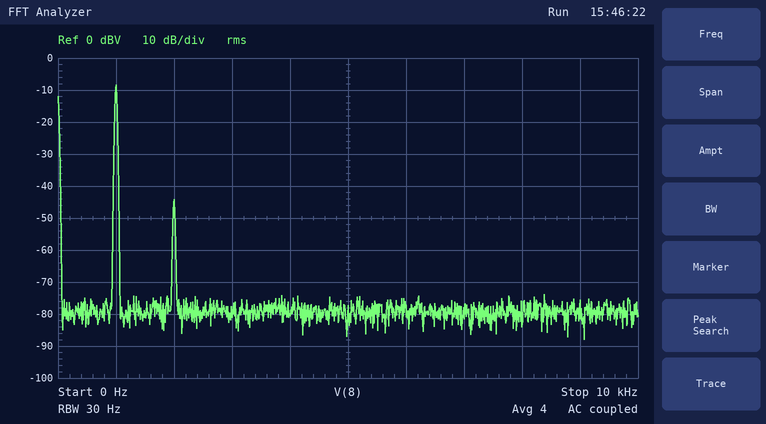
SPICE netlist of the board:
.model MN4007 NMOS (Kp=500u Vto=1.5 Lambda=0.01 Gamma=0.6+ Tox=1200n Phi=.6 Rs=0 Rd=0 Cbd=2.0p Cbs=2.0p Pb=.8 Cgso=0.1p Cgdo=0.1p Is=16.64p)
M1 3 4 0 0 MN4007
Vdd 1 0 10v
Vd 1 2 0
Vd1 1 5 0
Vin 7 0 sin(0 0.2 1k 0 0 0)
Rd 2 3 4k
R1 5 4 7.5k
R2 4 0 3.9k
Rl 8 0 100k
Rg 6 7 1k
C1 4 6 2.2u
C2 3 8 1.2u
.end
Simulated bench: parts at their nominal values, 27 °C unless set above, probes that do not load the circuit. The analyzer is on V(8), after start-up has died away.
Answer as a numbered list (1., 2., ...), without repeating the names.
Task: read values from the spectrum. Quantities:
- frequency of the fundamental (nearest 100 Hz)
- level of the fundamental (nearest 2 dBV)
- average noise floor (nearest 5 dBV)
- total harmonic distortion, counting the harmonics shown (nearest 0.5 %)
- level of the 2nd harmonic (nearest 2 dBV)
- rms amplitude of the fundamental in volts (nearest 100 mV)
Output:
1. 1.0 kHz
2. -8 dBV
3. -80 dBV
4. 1.5 %
5. -44 dBV
6. 400 mV
